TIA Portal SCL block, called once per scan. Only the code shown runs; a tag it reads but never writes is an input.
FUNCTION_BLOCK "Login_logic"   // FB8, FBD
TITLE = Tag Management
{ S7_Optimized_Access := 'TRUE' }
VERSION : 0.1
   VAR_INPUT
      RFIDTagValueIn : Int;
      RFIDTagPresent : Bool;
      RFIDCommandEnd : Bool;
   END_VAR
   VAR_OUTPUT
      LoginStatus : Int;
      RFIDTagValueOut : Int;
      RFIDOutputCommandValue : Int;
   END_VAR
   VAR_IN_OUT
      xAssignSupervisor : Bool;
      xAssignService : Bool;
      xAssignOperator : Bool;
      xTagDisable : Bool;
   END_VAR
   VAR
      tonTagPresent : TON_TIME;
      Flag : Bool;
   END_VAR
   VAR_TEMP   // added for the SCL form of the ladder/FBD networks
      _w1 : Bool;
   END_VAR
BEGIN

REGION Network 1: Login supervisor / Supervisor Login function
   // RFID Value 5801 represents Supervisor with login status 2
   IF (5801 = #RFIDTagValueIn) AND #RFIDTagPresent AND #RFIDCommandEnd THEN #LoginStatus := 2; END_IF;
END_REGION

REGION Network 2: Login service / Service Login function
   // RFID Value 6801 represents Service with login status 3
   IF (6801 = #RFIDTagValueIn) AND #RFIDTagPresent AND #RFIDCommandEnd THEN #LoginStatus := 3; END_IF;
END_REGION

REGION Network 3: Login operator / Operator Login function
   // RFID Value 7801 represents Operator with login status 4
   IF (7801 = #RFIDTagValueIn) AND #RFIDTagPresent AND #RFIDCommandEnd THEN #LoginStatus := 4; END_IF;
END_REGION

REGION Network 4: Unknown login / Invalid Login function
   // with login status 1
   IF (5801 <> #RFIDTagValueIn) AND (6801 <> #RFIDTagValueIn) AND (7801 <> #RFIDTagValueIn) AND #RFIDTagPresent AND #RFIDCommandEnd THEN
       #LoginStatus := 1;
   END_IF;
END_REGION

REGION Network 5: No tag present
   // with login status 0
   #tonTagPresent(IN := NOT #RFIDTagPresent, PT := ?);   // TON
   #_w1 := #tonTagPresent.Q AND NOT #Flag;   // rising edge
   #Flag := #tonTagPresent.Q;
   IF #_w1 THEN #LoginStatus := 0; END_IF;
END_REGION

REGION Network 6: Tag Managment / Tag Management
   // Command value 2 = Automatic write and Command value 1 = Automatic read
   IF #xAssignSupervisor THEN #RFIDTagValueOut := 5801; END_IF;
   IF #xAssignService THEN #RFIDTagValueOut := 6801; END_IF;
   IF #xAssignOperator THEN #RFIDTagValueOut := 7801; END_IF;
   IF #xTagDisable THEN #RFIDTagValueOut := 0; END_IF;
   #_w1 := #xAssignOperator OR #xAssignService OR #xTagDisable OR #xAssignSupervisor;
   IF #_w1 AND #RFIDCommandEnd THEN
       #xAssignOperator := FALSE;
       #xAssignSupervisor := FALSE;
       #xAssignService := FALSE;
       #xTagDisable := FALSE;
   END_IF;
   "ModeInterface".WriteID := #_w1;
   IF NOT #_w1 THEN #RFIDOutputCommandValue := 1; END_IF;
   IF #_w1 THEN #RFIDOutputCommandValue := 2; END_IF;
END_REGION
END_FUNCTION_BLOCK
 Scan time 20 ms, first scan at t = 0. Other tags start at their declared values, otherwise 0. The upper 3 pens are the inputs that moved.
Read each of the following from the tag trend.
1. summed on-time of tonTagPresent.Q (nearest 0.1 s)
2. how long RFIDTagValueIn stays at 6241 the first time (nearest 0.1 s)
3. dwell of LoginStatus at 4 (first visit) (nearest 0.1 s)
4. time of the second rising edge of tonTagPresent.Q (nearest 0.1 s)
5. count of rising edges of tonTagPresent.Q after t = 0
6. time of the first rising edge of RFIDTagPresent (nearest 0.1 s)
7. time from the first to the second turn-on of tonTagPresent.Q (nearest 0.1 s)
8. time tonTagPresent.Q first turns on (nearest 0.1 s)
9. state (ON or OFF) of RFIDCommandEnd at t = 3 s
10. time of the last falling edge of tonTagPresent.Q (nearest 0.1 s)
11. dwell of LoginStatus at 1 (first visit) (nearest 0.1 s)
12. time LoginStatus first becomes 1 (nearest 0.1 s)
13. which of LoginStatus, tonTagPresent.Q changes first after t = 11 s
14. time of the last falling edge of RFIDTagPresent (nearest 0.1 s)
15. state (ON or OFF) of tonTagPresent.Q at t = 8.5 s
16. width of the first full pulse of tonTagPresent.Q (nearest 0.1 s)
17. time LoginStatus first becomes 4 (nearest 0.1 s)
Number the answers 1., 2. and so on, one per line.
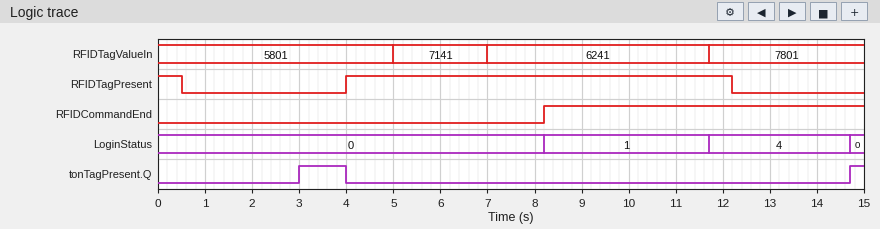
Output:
1. 1.3 s
2. 4.7 s
3. 3.0 s
4. 14.7 s
5. 2
6. 4.0 s
7. 11.7 s
8. 3.0 s
9. OFF
10. 4.0 s
11. 3.5 s
12. 8.2 s
13. LoginStatus
14. 12.2 s
15. OFF
16. 1.0 s
17. 11.7 s
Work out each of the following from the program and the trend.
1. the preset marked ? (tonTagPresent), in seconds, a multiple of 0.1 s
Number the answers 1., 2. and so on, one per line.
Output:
1. 2.5 s
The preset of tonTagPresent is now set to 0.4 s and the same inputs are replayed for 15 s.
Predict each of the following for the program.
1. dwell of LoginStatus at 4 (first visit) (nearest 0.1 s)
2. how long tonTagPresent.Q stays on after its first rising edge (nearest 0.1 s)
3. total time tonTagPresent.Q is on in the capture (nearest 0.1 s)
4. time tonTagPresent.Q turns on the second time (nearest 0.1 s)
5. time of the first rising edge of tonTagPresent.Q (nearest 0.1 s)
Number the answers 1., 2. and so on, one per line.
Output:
1. 0.9 s
2. 3.1 s
3. 5.5 s
4. 12.6 s
5. 0.9 s
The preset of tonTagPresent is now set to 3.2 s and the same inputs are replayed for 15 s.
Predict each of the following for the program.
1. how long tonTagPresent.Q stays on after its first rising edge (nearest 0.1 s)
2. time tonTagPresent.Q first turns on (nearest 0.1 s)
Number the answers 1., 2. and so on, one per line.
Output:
1. 0.3 s
2. 3.7 s
